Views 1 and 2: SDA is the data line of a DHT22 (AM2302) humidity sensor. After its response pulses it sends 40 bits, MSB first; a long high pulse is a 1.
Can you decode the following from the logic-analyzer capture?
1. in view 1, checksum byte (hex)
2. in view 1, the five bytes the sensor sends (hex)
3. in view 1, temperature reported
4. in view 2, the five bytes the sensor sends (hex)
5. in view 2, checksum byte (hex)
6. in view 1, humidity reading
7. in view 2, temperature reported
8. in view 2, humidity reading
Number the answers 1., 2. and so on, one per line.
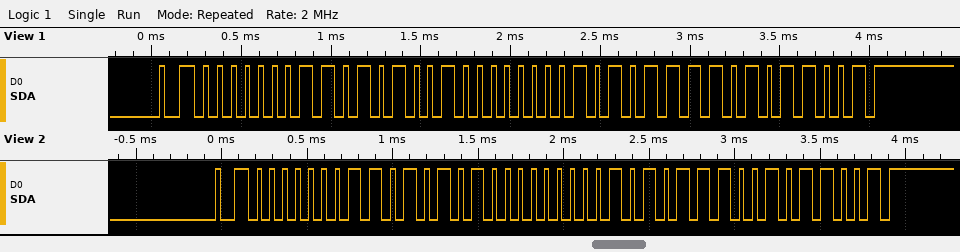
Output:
1. 0x59
2. 01 A9 00 AF 59
3. 17.5 °C
4. 01 AA 00 AE 59
5. 0x59
6. 42.5 %
7. 17.4 °C
8. 42.6 %
